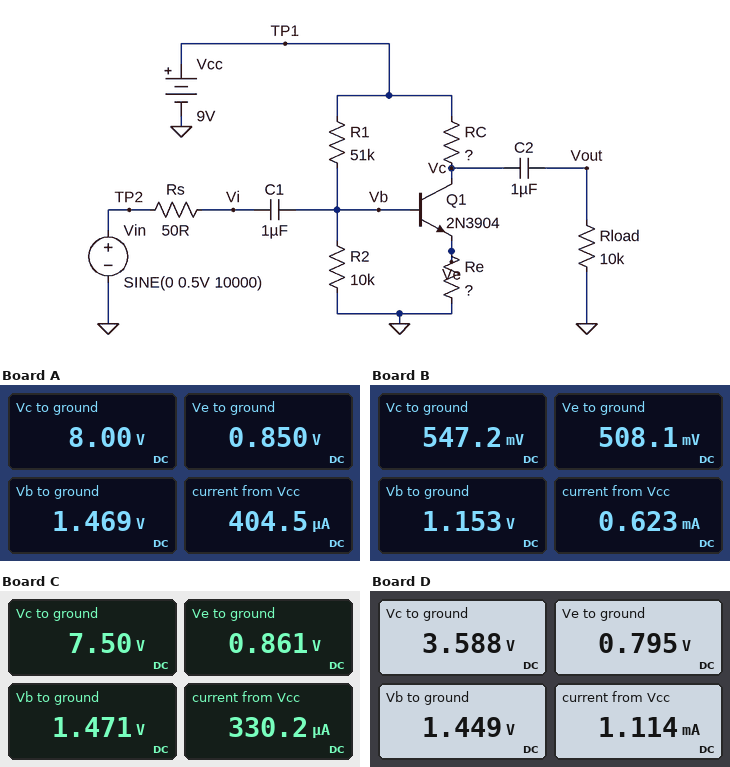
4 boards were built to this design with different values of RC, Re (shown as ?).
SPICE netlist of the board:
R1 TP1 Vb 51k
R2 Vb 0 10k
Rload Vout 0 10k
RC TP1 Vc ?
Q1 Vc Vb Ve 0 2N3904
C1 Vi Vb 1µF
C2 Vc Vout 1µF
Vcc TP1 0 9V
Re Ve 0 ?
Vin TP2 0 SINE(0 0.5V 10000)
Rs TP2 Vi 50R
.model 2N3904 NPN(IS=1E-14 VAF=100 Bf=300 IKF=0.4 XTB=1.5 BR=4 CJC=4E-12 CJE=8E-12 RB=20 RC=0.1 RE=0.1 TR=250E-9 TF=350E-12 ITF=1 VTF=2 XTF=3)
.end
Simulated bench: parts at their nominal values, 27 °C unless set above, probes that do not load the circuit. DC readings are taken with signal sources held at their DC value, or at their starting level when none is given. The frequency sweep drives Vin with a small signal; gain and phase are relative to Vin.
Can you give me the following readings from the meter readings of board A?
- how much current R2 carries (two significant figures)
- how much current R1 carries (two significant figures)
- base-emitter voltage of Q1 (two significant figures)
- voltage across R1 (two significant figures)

150 µA
150 µA
620 mV
7.5 V
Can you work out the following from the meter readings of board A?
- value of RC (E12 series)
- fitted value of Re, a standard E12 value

3.9 kΩ
3.3 kΩ
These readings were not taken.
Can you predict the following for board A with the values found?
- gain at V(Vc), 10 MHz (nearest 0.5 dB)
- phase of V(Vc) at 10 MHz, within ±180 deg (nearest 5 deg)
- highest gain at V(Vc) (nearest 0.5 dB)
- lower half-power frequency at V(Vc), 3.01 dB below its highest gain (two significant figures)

-1.5 dB
135 deg
0.5 dB
31 Hz
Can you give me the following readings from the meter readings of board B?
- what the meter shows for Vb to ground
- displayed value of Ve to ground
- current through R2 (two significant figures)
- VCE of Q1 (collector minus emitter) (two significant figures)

1.153 V
508.1 mV
120 µA
39 mV
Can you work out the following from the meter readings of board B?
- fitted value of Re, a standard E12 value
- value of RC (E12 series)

1 kΩ
18 kΩ
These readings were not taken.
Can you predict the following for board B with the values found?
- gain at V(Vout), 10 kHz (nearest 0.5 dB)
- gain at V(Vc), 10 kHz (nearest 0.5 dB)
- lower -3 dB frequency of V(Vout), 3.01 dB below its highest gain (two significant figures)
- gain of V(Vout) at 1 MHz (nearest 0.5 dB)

-9.0 dB
-9.0 dB
170 kHz
-1.0 dB
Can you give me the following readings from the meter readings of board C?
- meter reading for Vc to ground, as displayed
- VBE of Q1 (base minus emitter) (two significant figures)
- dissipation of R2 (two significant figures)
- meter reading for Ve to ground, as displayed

7.50 V
610 mV
220 µW
0.861 V
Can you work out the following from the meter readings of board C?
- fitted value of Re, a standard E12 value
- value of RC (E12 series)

4.7 kΩ
8.2 kΩ
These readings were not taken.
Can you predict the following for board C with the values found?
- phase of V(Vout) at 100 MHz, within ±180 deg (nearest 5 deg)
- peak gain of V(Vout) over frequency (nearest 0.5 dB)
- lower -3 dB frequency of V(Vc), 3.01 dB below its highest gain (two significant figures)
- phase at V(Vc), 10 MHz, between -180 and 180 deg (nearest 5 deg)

15 deg
0.5 dB
18 Hz
115 deg
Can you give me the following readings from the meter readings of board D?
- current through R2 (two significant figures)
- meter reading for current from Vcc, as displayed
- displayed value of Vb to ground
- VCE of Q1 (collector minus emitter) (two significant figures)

140 µA
1.114 mA
1.449 V
2.8 V
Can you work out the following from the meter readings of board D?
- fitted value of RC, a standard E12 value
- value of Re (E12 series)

5.6 kΩ
820 Ω
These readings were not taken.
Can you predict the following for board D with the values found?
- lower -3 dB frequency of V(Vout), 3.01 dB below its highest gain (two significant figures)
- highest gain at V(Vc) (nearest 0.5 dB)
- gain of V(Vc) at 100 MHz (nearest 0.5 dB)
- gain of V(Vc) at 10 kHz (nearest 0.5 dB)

24 Hz
12.5 dB
2.0 dB
12.5 dB
